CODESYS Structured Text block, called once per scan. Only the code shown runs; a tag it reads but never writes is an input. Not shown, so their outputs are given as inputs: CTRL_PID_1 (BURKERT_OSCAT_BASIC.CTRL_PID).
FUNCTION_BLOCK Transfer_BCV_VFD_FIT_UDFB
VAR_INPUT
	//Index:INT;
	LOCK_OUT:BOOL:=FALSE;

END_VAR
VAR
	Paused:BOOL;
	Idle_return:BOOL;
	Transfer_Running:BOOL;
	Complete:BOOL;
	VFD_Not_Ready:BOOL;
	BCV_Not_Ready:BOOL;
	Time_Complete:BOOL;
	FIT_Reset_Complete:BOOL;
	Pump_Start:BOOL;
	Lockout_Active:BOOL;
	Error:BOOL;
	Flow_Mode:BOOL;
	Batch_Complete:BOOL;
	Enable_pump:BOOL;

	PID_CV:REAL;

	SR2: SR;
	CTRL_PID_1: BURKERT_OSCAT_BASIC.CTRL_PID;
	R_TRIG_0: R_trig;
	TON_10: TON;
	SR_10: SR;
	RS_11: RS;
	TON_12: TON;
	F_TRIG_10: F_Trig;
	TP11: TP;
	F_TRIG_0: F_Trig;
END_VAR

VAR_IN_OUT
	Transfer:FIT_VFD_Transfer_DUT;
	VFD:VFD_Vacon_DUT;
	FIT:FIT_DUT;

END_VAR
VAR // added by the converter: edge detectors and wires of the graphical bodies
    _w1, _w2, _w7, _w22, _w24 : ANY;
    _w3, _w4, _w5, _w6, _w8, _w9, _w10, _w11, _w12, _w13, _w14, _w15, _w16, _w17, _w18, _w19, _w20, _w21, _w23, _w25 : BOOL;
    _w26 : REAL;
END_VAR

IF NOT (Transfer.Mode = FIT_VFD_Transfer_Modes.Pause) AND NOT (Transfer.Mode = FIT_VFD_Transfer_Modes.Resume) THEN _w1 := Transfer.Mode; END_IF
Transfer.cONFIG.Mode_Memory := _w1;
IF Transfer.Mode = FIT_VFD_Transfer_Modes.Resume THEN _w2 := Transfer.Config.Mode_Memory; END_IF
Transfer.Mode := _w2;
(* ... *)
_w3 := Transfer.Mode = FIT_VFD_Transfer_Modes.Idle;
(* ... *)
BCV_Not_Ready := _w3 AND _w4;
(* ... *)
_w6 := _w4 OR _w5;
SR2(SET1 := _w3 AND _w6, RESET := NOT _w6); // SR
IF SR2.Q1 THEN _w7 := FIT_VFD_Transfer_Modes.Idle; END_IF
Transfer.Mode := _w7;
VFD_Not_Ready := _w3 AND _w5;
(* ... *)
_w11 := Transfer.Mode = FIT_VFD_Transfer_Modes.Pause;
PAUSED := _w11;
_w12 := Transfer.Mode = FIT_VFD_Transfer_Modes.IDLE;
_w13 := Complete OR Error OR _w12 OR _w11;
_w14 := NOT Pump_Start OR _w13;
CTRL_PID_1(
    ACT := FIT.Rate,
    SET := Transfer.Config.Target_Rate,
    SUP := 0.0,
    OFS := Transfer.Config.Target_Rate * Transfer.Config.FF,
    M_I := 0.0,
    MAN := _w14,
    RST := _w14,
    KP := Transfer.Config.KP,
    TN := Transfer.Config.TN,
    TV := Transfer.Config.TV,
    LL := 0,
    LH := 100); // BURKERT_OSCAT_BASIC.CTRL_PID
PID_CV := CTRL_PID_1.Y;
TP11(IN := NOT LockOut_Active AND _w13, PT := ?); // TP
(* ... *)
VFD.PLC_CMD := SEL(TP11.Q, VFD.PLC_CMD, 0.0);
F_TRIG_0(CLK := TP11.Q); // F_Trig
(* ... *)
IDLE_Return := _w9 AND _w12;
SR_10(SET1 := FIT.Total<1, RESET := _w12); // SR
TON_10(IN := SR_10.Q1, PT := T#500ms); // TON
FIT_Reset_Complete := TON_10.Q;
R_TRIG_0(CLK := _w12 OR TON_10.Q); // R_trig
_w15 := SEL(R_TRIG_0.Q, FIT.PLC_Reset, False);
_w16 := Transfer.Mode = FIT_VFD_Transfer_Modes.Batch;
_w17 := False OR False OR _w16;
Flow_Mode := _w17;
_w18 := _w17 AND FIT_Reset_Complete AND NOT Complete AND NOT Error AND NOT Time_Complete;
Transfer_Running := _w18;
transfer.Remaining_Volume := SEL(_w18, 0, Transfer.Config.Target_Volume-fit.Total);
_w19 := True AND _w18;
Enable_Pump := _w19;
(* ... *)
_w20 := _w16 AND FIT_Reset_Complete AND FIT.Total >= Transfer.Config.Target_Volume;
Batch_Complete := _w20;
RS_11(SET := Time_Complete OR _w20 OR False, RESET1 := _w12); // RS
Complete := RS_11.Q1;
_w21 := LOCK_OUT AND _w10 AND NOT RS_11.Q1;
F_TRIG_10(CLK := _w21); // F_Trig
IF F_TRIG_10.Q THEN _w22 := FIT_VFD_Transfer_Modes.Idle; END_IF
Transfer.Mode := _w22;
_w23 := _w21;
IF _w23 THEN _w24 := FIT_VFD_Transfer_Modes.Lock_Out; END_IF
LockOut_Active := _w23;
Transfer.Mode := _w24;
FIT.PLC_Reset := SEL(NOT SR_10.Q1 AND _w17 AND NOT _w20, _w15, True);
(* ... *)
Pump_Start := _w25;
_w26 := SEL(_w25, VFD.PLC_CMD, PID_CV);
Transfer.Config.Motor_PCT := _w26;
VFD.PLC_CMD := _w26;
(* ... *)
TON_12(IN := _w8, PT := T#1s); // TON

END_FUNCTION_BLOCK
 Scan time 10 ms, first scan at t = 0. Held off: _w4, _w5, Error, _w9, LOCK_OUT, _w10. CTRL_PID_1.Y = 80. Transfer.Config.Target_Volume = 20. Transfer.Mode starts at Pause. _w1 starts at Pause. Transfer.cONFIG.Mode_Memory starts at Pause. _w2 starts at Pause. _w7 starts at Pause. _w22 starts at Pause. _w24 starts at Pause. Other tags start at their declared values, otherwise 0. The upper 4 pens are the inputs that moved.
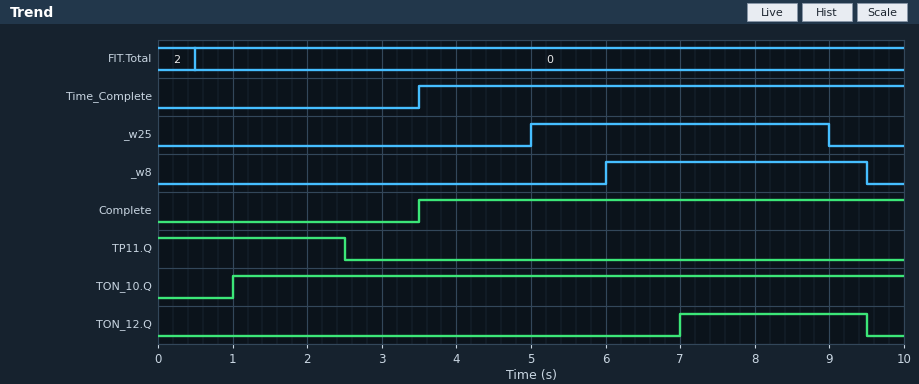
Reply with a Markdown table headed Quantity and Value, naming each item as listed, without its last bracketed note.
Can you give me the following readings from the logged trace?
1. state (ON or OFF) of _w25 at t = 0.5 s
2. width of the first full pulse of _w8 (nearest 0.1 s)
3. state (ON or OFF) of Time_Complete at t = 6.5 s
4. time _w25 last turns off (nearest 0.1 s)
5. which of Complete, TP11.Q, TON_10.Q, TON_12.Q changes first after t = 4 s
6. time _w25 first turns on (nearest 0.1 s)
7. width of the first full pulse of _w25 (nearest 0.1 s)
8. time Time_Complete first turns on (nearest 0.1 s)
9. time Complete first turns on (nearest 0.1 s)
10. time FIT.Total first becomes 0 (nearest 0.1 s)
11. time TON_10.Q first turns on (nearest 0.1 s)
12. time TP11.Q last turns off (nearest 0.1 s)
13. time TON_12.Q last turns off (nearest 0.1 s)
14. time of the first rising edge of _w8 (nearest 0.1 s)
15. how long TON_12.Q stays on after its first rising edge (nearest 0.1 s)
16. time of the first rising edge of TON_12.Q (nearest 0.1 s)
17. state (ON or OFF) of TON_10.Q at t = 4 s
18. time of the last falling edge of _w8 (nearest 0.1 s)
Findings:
| Quantity | Value |
|---|---|
| state (ON or OFF) of _w25 at t = 0.5 s | OFF |
| width of the first full pulse of _w8 | 3.5 s |
| state (ON or OFF) of Time_Complete at t = 6.5 s | ON |
| time _w25 last turns off | 9.0 s |
| which of Complete, TP11.Q, TON_10.Q, TON_12.Q changes first after t = 4 s | TON_12.Q |
| time _w25 first turns on | 5.0 s |
| width of the first full pulse of _w25 | 4.0 s |
| time Time_Complete first turns on | 3.5 s |
| time Complete first turns on | 3.5 s |
| time FIT.Total first becomes 0 | 0.5 s |
| time TON_10.Q first turns on | 1.0 s |
| time TP11.Q last turns off | 2.5 s |
| time TON_12.Q last turns off | 9.5 s |
| time of the first rising edge of _w8 | 6.0 s |
| how long TON_12.Q stays on after its first rising edge | 2.5 s |
| time of the first rising edge of TON_12.Q | 7.0 s |
| state (ON or OFF) of TON_10.Q at t = 4 s | ON |
| time of the last falling edge of _w8 | 9.5 s |
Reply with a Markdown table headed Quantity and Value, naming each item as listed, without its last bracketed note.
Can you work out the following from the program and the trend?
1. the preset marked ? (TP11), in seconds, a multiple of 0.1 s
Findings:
| Quantity | Value |
|---|---|
| the preset marked ? (TP11), in seconds, a multiple of 0.1 s | 2.5 s |
